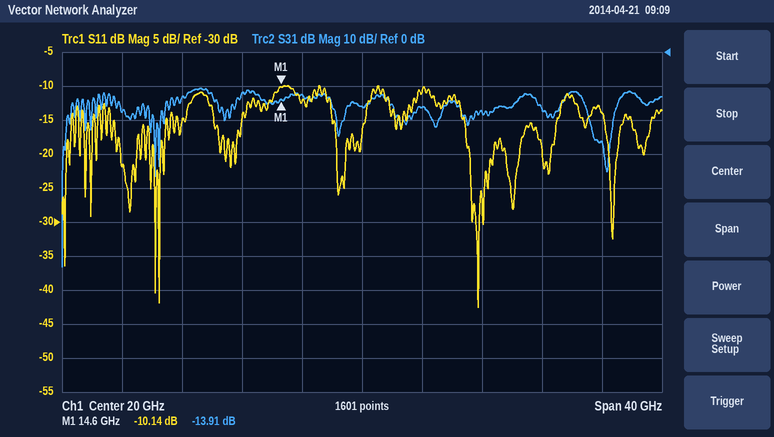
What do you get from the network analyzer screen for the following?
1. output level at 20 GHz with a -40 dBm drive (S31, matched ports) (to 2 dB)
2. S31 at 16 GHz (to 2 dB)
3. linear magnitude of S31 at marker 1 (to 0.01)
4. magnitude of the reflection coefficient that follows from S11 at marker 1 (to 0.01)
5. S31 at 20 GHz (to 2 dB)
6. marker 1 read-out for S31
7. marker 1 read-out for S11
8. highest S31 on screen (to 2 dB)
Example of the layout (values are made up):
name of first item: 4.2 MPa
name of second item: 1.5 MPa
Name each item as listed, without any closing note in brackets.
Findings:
output level at 20 GHz with a -40 dBm drive (S31, matched ports): -56 dBm
S31 at 16 GHz: -12 dB
linear magnitude of S31 at marker 1: 0.20
magnitude of the reflection coefficient that follows from S11 at marker 1: 0.31
S31 at 20 GHz: -16 dB
marker 1 read-out for S31: -13.91 dB
marker 1 read-out for S11: -10.14 dB
highest S31 on screen: -10 dB
